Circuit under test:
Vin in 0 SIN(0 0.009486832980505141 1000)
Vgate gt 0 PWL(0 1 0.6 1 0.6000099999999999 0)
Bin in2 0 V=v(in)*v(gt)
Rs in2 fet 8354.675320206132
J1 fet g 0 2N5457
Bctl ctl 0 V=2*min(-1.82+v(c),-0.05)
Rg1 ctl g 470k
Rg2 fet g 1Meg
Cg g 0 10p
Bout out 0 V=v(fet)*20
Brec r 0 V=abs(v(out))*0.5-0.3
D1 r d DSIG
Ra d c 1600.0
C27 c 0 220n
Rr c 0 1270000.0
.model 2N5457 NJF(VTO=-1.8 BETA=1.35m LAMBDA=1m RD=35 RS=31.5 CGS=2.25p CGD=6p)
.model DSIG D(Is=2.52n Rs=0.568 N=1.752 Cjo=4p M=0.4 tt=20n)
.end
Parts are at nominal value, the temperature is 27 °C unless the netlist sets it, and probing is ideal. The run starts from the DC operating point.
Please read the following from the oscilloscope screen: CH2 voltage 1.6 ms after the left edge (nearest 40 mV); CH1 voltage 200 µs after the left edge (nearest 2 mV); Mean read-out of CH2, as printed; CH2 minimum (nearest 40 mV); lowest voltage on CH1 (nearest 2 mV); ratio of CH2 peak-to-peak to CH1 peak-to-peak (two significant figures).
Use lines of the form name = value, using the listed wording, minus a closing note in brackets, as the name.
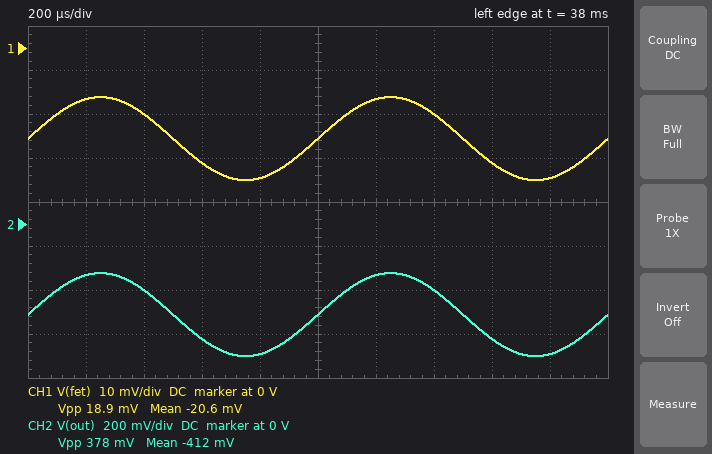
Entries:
CH2 voltage 1.6 ms after the left edge = -520 mV
CH1 voltage 200 µs after the left edge = -12 mV
Mean read-out of CH2, as printed = -412 mV
CH2 minimum = -600 mV
lowest voltage on CH1 = -30 mV
ratio of CH2 peak-to-peak to CH1 peak-to-peak = 20
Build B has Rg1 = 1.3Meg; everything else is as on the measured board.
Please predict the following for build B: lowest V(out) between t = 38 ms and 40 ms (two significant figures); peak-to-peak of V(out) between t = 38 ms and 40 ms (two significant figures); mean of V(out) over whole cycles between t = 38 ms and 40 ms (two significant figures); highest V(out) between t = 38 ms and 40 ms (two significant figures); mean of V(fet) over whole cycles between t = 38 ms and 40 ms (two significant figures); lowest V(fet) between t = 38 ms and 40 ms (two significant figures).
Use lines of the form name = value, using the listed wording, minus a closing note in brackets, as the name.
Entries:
lowest V(out) between t = 38 ms and 40 ms = -80 mV
peak-to-peak of V(out) between t = 38 ms and 40 ms = 67 mV
mean of V(out) over whole cycles between t = 38 ms and 40 ms = -47 mV
highest V(out) between t = 38 ms and 40 ms = -13 mV
mean of V(fet) over whole cycles between t = 38 ms and 40 ms = -2.3 mV
lowest V(fet) between t = 38 ms and 40 ms = -4.0 mV
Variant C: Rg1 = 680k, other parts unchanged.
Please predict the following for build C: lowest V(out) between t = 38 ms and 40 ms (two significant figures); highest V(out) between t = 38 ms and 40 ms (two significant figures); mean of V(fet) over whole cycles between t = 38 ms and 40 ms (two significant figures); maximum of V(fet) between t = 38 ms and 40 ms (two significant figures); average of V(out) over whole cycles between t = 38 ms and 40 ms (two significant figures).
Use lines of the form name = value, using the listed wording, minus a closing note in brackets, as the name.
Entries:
lowest V(out) between t = 38 ms and 40 ms = -550 mV
highest V(out) between t = 38 ms and 40 ms = -170 mV
mean of V(fet) over whole cycles between t = 38 ms and 40 ms = -18 mV
maximum of V(fet) between t = 38 ms and 40 ms = -8.6 mV
average of V(out) over whole cycles between t = 38 ms and 40 ms = -360 mV
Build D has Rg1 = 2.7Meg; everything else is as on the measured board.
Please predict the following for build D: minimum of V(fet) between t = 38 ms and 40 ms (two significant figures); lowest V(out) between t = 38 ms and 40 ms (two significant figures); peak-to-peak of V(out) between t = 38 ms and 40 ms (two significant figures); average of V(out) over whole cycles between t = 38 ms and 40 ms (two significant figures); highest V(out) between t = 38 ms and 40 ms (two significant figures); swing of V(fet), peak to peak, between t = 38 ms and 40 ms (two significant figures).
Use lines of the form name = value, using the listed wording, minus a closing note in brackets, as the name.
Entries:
minimum of V(fet) between t = 38 ms and 40 ms = -1.0 mV
lowest V(out) between t = 38 ms and 40 ms = -21 mV
peak-to-peak of V(out) between t = 38 ms and 40 ms = 22 mV
average of V(out) over whole cycles between t = 38 ms and 40 ms = -9.7 mV
highest V(out) between t = 38 ms and 40 ms = 1.5 mV
swing of V(fet), peak to peak, between t = 38 ms and 40 ms = 1.1 mV
